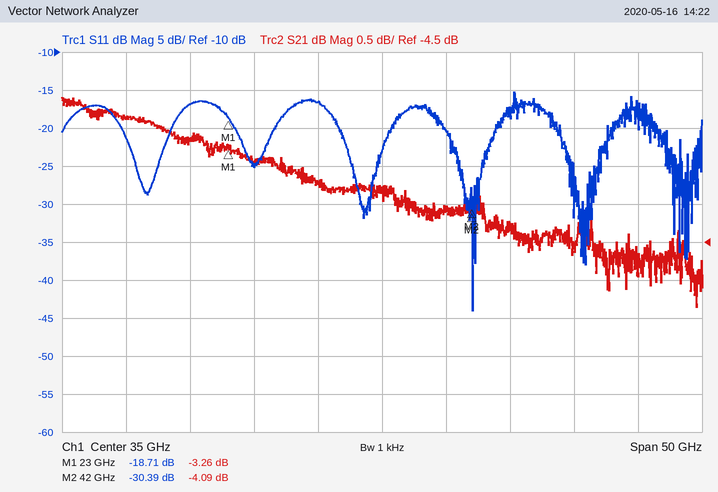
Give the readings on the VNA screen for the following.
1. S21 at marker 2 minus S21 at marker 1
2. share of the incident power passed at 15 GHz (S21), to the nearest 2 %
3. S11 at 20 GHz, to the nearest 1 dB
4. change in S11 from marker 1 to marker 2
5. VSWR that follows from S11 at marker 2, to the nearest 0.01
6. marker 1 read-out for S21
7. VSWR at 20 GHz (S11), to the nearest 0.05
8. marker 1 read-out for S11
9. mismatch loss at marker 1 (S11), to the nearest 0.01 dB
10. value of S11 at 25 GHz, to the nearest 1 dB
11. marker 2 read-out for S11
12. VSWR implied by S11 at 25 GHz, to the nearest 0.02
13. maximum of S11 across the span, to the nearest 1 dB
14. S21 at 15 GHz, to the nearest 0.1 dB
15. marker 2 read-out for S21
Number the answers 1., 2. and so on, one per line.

1. -0.83 dB
2. 52 %
3. -17 dB
4. -11.68 dB
5. 1.06
6. -3.26 dB
7. 1.35
8. -18.71 dB
9. 0.06 dB
10. -25 dB
11. -30.39 dB
12. 1.12
13. -15 dB
14. -2.9 dB
15. -4.09 dB
